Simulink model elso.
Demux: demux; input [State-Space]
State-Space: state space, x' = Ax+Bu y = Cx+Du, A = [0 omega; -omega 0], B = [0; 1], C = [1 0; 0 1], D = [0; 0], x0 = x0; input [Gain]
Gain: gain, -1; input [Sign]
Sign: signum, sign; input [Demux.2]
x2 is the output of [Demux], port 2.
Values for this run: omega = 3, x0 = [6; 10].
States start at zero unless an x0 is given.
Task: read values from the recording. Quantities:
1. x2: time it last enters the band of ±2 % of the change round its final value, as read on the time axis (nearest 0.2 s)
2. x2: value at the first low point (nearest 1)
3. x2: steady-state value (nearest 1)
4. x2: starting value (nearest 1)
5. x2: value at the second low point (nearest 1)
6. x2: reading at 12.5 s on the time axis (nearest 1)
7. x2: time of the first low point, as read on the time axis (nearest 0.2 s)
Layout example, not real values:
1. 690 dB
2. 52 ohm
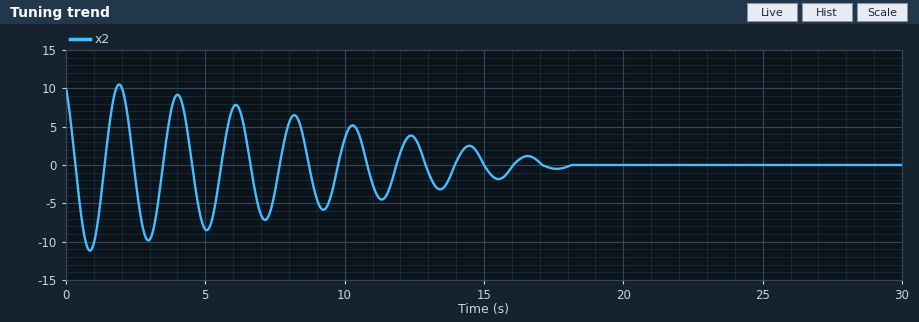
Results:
1. 18.0 s
2. -11
3. 0
4. 10
5. -10
6. 4
7. 0.8 s
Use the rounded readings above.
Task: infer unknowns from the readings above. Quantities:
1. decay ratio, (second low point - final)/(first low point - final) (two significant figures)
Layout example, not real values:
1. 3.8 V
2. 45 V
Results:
1. 0.91
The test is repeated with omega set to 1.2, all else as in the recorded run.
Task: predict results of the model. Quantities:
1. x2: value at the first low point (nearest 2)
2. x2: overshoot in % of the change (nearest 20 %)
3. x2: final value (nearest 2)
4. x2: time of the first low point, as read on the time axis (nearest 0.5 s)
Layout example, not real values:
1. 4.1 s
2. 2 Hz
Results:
1. -10
2. 100 %
3. 0
4. 2.0 s
